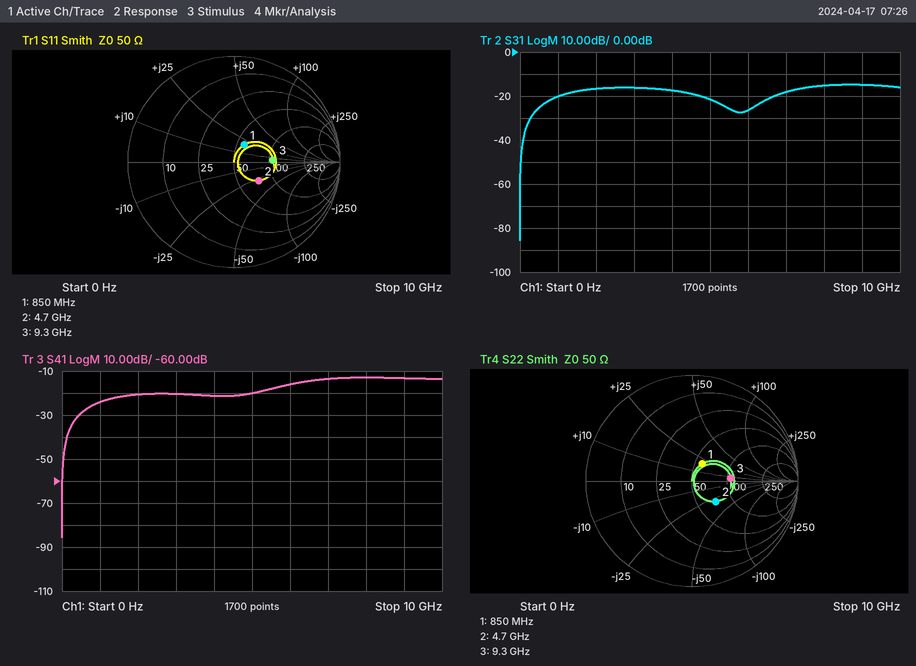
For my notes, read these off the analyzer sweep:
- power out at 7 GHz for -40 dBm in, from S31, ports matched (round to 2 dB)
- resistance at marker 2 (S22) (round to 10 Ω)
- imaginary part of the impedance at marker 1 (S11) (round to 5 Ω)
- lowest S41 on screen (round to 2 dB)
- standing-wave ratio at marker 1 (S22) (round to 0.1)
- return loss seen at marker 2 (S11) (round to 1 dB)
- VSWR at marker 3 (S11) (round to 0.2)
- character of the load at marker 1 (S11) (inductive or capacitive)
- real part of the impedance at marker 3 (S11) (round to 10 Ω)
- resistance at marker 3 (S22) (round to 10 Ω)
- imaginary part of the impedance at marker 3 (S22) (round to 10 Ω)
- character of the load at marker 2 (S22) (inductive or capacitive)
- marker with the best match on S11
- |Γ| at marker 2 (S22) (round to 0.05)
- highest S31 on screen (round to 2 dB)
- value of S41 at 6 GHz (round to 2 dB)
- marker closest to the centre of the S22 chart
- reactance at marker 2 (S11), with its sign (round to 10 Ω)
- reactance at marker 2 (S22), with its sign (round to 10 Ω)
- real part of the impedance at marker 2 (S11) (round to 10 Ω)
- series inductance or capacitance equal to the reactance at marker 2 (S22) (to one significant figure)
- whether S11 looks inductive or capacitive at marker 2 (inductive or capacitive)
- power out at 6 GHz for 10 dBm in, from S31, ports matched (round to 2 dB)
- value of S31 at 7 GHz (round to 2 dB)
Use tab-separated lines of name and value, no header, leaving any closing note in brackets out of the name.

power out at 7 GHz for -40 dBm in, from S31, ports matched	-58 dBm
resistance at marker 2 (S22)	70 Ω
imaginary part of the impedance at marker 1 (S11)	+20 Ω
lowest S41 on screen	-86 dB
standing-wave ratio at marker 1 (S22)	1.5
return loss seen at marker 2 (S11)	11 dB
VSWR at marker 3 (S11)	2.2
character of the load at marker 1 (S11)	inductive
real part of the impedance at marker 3 (S11)	110 Ω
resistance at marker 3 (S22)	110 Ω
imaginary part of the impedance at marker 3 (S22)	+10 Ω
character of the load at marker 2 (S22)	capacitive
marker with the best match on S11	marker 1
|Γ| at marker 2 (S22)	0.30
highest S31 on screen	-14 dB
value of S41 at 6 GHz	-16 dB
marker closest to the centre of the S22 chart	marker 1
reactance at marker 2 (S11), with its sign	-30 Ω
reactance at marker 2 (S22), with its sign	-30 Ω
real part of the impedance at marker 2 (S11)	70 Ω
series inductance or capacitance equal to the reactance at marker 2 (S22)	1 pF
whether S11 looks inductive or capacitive at marker 2	capacitive
power out at 6 GHz for 10 dBm in, from S31, ports matched	-16 dBm
value of S31 at 7 GHz	-18 dB
